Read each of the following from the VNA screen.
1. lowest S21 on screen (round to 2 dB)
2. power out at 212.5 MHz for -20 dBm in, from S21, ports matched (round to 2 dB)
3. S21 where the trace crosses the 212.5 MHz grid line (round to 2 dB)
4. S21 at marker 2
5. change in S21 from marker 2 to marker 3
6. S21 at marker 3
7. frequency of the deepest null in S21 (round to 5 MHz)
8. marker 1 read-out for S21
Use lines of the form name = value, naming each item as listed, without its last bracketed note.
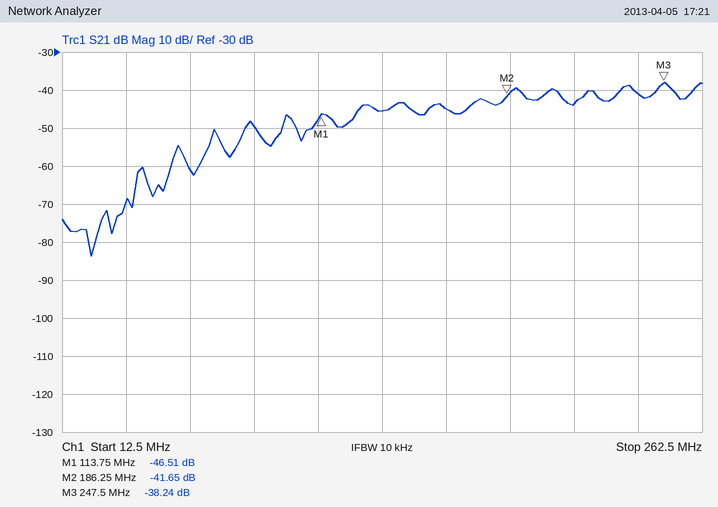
lowest S21 on screen = -84 dB
power out at 212.5 MHz for -20 dBm in, from S21, ports matched = -64 dBm
S21 where the trace crosses the 212.5 MHz grid line = -44 dB
S21 at marker 2 = -41.65 dB
change in S21 from marker 2 to marker 3 = 3.41 dB
S21 at marker 3 = -38.24 dB
frequency of the deepest null in S21 = 25 MHz
marker 1 read-out for S21 = -46.51 dB
